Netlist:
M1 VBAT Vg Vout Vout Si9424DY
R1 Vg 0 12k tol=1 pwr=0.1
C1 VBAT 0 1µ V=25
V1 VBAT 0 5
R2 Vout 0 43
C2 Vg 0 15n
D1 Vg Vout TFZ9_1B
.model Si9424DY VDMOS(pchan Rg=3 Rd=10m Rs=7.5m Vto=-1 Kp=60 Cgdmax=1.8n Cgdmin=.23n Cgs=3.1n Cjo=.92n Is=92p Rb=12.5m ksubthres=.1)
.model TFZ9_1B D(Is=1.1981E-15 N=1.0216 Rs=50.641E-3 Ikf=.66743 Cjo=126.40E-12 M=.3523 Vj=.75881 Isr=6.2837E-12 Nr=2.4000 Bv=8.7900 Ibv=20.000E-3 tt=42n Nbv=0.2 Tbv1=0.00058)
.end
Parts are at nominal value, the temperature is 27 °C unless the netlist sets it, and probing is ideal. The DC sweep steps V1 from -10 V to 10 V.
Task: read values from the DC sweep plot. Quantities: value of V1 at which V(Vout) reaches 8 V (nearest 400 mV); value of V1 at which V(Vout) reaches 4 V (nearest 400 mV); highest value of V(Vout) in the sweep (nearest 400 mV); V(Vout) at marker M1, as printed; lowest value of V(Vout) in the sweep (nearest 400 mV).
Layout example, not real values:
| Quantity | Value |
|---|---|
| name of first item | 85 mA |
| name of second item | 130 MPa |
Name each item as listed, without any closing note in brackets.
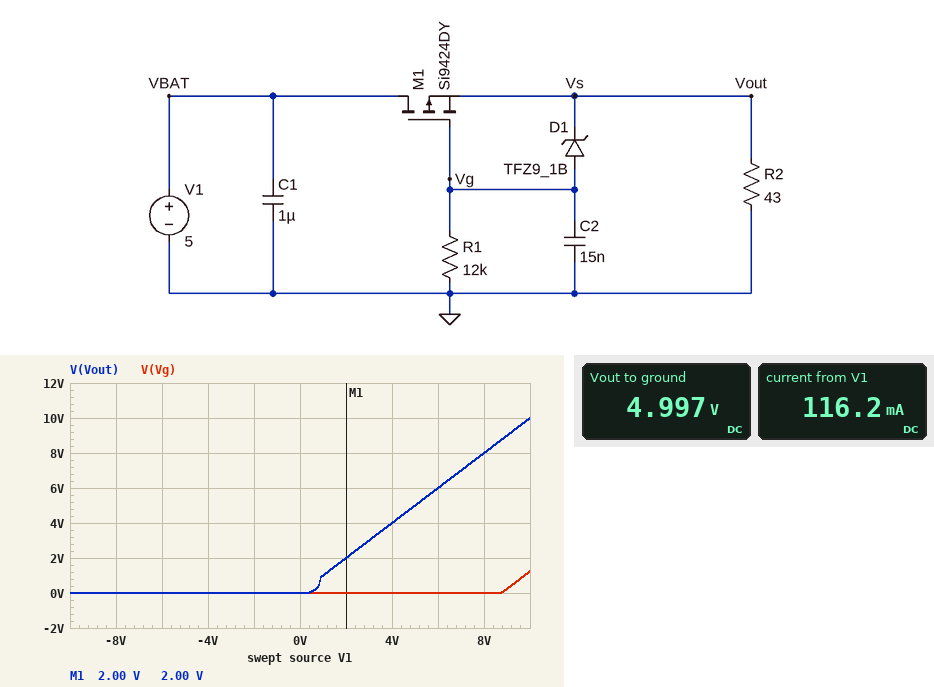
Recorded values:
| Quantity | Value |
|---|---|
| value of V1 at which V(Vout) reaches 8 V | 8.0 V |
| value of V1 at which V(Vout) reaches 4 V | 4.0 V |
| highest value of V(Vout) in the sweep | 10.0 V |
| V(Vout) at marker M1, as printed | 2.00 V |
| lowest value of V(Vout) in the sweep | 0 V |
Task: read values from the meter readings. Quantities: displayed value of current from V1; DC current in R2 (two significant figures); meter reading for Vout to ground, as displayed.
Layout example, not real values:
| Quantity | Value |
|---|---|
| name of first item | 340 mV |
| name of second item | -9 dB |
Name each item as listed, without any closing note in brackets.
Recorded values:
| Quantity | Value |
|---|---|
| displayed value of current from V1 | 116.2 mA |
| DC current in R2 | 120 mA |
| meter reading for Vout to ground, as displayed | 4.997 V |
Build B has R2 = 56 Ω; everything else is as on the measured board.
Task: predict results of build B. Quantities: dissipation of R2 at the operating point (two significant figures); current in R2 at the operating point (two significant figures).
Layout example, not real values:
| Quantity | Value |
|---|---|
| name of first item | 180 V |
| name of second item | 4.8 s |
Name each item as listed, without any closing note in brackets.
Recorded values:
| Quantity | Value |
|---|---|
| dissipation of R2 at the operating point | 450 mW |
| current in R2 at the operating point | 89 mA |
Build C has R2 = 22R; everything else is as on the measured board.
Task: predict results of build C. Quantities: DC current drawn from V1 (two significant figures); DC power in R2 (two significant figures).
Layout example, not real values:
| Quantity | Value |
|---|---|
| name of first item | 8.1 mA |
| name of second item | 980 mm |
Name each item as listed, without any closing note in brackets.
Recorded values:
| Quantity | Value |
|---|---|
| DC current drawn from V1 | 230 mA |
| DC power in R2 | 1.1 W |
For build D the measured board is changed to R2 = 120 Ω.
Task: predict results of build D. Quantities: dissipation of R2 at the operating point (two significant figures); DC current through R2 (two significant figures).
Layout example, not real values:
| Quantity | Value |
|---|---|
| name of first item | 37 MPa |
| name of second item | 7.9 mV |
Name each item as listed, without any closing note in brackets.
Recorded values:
| Quantity | Value |
|---|---|
| dissipation of R2 at the operating point | 210 mW |
| DC current through R2 | 42 mA |
